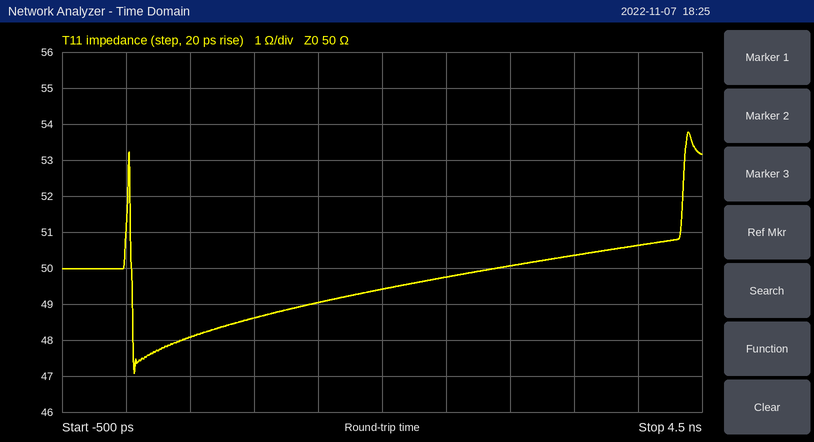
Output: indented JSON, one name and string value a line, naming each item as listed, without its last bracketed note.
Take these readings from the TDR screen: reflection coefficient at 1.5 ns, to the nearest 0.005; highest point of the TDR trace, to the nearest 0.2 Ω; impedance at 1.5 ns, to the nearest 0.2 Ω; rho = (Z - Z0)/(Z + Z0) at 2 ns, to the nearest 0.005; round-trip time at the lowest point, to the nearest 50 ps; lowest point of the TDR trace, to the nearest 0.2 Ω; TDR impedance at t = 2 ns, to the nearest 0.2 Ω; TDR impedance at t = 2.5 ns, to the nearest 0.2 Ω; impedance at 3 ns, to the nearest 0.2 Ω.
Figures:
{
  "reflection coefficient at 1.5 ns, to the nearest 0.005": "-0.010",
  "highest point of the TDR trace, to the nearest 0.2 Ω": "53.8 Ω",
  "impedance at 1.5 ns, to the nearest 0.2 Ω": "49.0 Ω",
  "rho = (Z - Z0)/(Z + Z0) at 2 ns, to the nearest 0.005": "-0.005",
  "round-trip time at the lowest point, to the nearest 50 ps": "50 ps",
  "lowest point of the TDR trace, to the nearest 0.2 Ω": "47.0 Ω",
  "TDR impedance at t = 2 ns, to the nearest 0.2 Ω": "49.4 Ω",
  "TDR impedance at t = 2.5 ns, to the nearest 0.2 Ω": "49.8 Ω",
  "impedance at 3 ns, to the nearest 0.2 Ω": "50.0 Ω"
}
